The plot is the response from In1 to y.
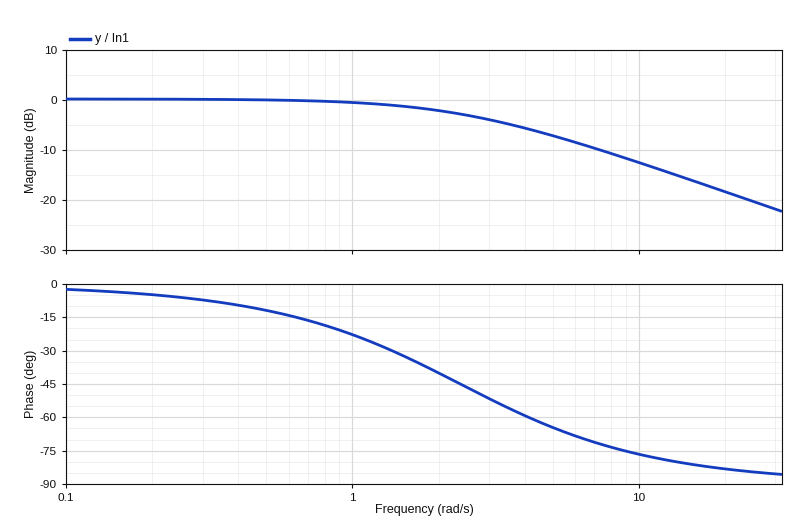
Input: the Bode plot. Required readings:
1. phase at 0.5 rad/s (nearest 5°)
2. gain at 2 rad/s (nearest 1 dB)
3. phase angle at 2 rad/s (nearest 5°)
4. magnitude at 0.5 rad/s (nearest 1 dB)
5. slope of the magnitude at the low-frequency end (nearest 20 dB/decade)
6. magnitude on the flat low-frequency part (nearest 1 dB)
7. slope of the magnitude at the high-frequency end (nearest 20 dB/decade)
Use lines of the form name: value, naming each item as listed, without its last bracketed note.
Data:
phase at 0.5 rad/s: -10°
gain at 2 rad/s: -2 dB
phase angle at 2 rad/s: -40°
magnitude at 0.5 rad/s: 0 dB
slope of the magnitude at the low-frequency end: 0 dB/decade
magnitude on the flat low-frequency part: 0 dB
slope of the magnitude at the high-frequency end: -20 dB/decade
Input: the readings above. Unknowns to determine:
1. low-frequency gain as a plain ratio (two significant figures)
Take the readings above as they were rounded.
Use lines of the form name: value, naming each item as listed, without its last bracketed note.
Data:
low-frequency gain as a plain ratio: 1.0
